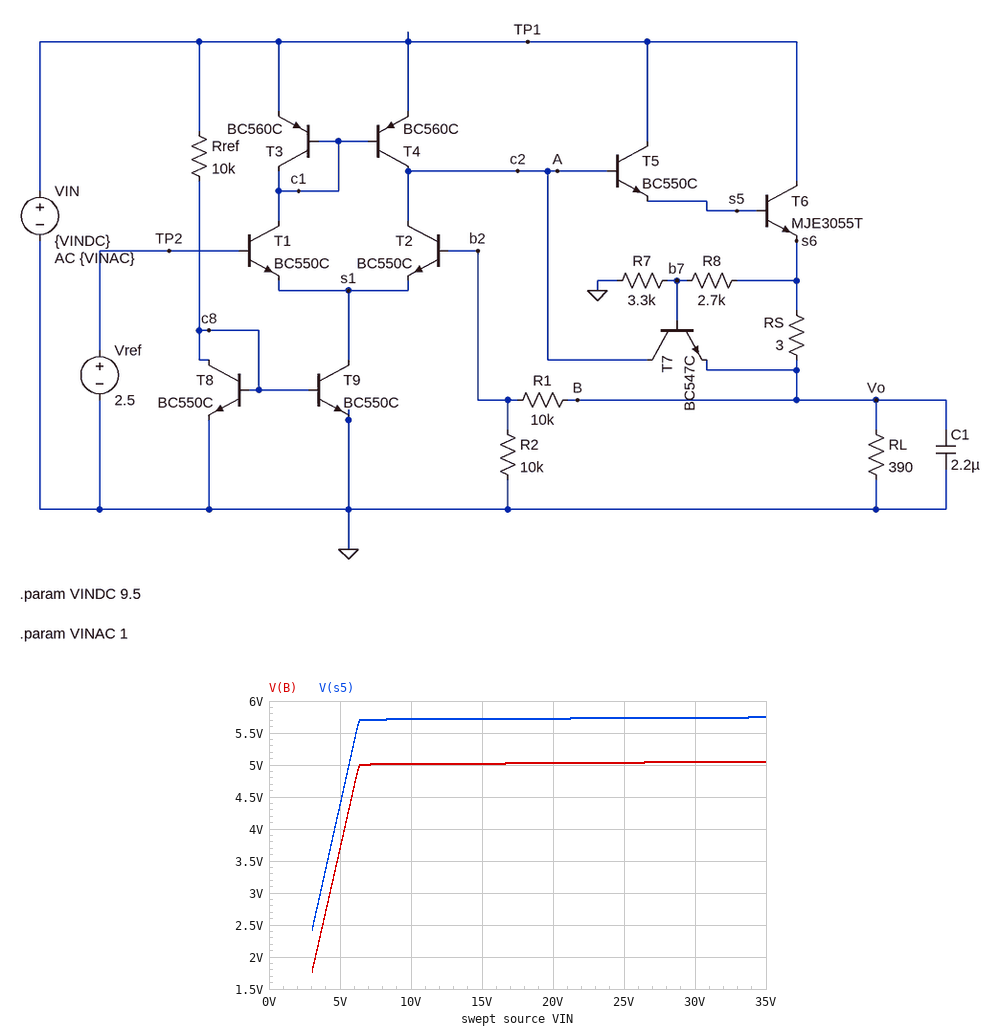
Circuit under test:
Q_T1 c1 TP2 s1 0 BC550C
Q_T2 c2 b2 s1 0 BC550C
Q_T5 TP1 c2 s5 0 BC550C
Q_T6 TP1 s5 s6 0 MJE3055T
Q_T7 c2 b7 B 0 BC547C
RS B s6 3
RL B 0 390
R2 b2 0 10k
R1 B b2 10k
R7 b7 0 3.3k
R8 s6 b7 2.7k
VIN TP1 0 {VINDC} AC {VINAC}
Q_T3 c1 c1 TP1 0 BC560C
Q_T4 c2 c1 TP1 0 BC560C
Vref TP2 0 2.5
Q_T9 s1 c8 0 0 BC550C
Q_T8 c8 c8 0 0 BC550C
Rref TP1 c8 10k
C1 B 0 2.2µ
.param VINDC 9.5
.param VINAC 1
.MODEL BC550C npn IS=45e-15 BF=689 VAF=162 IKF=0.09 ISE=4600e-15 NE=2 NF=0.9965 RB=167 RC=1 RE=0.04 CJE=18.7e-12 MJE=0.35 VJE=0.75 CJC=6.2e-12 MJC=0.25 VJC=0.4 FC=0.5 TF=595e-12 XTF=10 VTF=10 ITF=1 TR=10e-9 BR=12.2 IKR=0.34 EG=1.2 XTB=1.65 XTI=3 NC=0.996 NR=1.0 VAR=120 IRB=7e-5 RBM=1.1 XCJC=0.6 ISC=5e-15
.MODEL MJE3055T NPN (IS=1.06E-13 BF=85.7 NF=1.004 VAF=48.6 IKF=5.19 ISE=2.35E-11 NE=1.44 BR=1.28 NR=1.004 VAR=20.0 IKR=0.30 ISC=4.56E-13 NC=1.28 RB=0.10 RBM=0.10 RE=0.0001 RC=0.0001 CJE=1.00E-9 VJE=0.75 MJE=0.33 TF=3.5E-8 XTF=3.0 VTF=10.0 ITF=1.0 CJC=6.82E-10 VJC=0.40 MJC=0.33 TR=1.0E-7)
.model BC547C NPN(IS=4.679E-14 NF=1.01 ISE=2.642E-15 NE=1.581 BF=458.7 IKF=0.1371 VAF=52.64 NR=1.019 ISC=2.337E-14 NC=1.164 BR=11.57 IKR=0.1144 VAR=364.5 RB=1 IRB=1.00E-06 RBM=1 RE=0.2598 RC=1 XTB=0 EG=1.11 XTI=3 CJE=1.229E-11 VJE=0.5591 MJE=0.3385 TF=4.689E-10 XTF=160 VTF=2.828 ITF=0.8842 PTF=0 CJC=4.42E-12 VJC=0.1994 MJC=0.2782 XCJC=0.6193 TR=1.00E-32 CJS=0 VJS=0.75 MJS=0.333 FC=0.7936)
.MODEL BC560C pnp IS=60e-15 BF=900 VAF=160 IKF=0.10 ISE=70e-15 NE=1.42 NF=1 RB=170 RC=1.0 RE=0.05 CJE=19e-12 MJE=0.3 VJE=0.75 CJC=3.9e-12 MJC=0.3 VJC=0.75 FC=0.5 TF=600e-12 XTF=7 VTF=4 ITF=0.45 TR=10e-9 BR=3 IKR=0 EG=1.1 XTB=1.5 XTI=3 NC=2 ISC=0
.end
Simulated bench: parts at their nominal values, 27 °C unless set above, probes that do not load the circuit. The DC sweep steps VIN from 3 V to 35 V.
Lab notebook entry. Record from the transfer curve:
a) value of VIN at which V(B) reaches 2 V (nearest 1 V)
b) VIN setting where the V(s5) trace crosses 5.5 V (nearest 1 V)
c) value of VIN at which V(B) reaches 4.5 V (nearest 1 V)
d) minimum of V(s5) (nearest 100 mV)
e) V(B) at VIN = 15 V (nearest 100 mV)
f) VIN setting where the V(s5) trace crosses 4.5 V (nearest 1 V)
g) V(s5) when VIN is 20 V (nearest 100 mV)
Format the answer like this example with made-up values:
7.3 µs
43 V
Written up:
3 V
6 V
6 V
2.4 V
5.0 V
5 V
5.7 V
